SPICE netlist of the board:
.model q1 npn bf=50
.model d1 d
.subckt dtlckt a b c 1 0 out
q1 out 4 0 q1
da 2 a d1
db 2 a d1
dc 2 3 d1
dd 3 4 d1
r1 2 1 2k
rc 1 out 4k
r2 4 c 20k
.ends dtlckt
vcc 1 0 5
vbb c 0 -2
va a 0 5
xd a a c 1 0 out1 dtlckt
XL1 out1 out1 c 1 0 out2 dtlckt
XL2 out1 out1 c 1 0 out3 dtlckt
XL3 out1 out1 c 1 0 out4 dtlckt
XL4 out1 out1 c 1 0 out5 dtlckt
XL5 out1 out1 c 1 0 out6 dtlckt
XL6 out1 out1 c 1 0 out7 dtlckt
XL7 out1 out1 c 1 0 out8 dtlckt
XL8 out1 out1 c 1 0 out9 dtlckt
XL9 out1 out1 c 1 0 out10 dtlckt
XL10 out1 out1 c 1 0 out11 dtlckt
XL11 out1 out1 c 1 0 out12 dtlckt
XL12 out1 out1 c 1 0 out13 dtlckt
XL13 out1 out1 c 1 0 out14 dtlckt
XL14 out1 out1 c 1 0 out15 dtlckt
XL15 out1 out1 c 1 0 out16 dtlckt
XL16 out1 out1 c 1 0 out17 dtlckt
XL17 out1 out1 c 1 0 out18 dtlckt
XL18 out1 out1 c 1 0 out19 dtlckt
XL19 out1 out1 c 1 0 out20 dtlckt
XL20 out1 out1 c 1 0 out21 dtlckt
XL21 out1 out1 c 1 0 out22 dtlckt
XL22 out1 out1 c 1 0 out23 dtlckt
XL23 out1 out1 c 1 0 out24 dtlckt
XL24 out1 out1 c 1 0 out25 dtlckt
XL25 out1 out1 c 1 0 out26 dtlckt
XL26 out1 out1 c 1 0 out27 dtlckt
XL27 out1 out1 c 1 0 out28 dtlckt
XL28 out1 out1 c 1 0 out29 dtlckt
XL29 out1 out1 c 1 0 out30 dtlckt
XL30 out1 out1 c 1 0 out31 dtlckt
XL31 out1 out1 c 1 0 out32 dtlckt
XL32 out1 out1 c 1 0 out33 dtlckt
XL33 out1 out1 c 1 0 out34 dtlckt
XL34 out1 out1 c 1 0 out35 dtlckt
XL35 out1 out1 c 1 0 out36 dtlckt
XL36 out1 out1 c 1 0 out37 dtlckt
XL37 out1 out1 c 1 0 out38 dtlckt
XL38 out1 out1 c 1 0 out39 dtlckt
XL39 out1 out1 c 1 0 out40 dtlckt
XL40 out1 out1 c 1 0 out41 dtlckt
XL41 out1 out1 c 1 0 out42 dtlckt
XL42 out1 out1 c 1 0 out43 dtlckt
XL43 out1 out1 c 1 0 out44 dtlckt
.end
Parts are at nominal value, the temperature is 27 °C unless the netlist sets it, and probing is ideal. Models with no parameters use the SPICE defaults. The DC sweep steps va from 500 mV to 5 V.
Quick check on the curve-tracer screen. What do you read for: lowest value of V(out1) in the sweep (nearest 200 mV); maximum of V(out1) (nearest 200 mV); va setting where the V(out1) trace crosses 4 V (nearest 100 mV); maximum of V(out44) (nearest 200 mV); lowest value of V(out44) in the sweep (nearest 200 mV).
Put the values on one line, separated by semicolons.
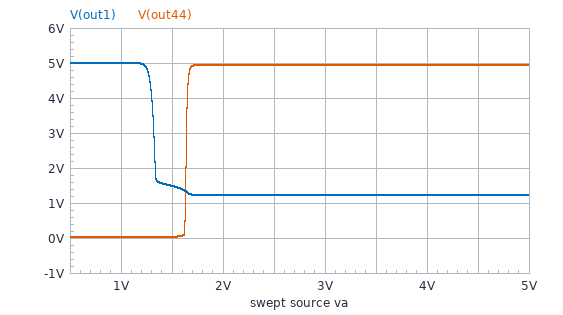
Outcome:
1.2 V; 5.0 V; 1.3 V; 5.0 V; 0 V
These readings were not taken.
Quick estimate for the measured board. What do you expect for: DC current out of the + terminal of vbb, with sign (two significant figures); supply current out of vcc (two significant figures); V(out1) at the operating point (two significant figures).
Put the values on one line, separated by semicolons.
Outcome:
-5.9 mA; 70 mA; 1.2 V
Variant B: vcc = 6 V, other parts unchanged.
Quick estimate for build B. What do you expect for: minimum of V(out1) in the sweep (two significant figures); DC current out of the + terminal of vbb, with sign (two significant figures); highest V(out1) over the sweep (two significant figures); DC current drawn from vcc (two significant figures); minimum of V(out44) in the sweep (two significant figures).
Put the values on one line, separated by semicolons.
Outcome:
1.1 V; -5.6 mA; 6.0 V; 94 mA; 27 mV
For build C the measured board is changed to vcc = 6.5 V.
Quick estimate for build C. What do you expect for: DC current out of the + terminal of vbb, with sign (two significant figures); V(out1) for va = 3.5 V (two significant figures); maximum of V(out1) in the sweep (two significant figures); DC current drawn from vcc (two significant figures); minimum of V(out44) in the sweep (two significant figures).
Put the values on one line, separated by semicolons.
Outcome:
-5.5 mA; 1.0 V; 6.5 V; 110 mA; 27 mV
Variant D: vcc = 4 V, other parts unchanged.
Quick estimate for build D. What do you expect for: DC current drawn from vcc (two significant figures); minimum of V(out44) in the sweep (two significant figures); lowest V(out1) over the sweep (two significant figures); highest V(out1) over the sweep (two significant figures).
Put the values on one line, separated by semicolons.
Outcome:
59 mA; 31 mV; 1.3 V; 4.0 V
